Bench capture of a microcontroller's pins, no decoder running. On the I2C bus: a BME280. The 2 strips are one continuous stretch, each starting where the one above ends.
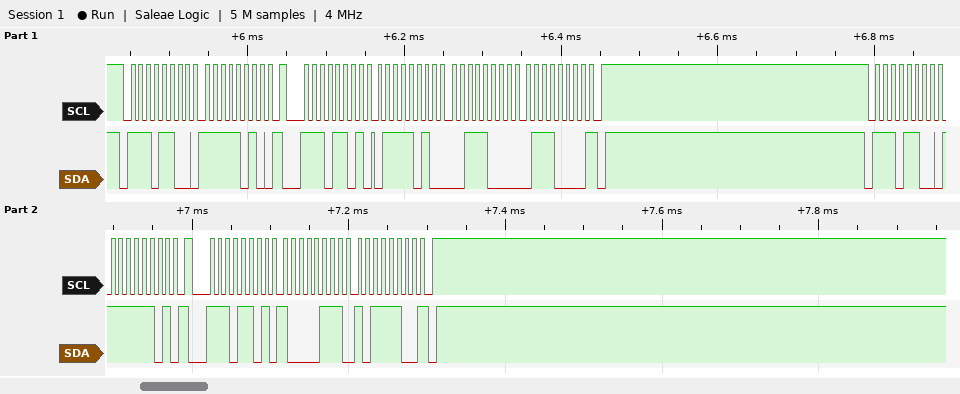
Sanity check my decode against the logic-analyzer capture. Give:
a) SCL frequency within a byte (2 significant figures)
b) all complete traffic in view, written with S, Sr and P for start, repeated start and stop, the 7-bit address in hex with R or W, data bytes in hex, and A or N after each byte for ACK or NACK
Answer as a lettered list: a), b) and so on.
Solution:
a) 100 kHz
b) S 76W A FA A Sr 76R A 7A A 38 A 70 N P S 76W A FD A Sr 76R A 87 A BC N P
